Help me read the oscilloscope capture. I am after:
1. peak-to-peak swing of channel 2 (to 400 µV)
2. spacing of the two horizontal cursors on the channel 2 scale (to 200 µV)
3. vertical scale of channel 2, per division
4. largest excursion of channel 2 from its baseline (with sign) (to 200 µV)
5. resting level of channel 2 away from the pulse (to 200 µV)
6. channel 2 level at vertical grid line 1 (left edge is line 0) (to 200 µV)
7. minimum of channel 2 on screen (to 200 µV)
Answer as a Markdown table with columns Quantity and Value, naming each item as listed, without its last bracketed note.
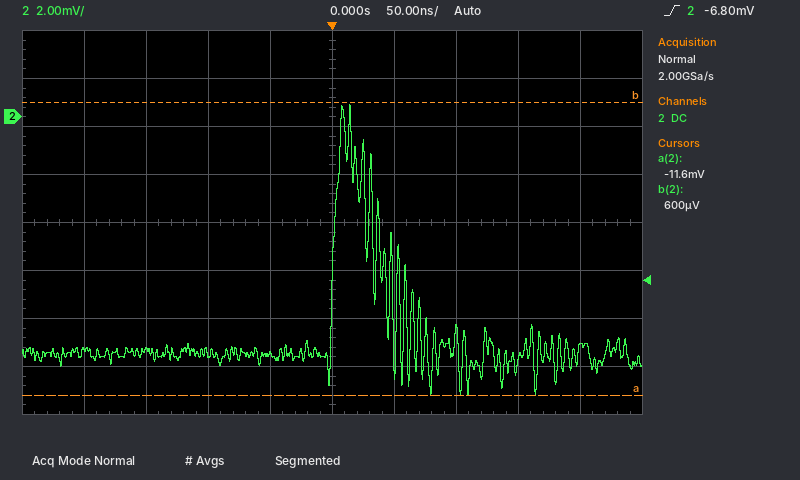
| Quantity | Value |
|---|---|
| peak-to-peak swing of channel 2 | 12.0 mV |
| spacing of the two horizontal cursors on the channel 2 scale | 12.2 mV |
| vertical scale of channel 2, per division | 2 mV |
| largest excursion of channel 2 from its baseline (with sign) | +10.4 mV |
| resting level of channel 2 away from the pulse | -9.8 mV |
| channel 2 level at vertical grid line 1 (left edge is line 0) | -9.8 mV |
| minimum of channel 2 on screen | -11.6 mV |
